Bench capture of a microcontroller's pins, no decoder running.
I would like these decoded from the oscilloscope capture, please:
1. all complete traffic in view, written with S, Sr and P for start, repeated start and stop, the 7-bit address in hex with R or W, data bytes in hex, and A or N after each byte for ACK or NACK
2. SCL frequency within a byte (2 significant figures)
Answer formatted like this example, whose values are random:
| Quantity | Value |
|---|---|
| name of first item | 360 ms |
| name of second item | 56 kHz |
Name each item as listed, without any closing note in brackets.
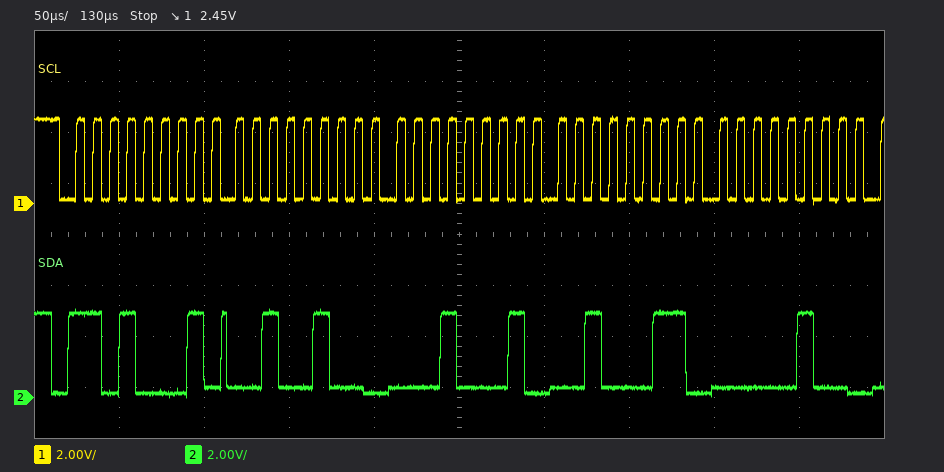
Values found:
| Quantity | Value |
|---|---|
| all complete traffic in view, written with S, Sr and P for start, repeated start and stop, the 7-bit address in hex with R or W, data bytes in hex, and A or N after each byte for ACK or NACK | S 68R A 24 A 11 A 23 A 04 A |
| SCL frequency within a byte | 100 kHz |
